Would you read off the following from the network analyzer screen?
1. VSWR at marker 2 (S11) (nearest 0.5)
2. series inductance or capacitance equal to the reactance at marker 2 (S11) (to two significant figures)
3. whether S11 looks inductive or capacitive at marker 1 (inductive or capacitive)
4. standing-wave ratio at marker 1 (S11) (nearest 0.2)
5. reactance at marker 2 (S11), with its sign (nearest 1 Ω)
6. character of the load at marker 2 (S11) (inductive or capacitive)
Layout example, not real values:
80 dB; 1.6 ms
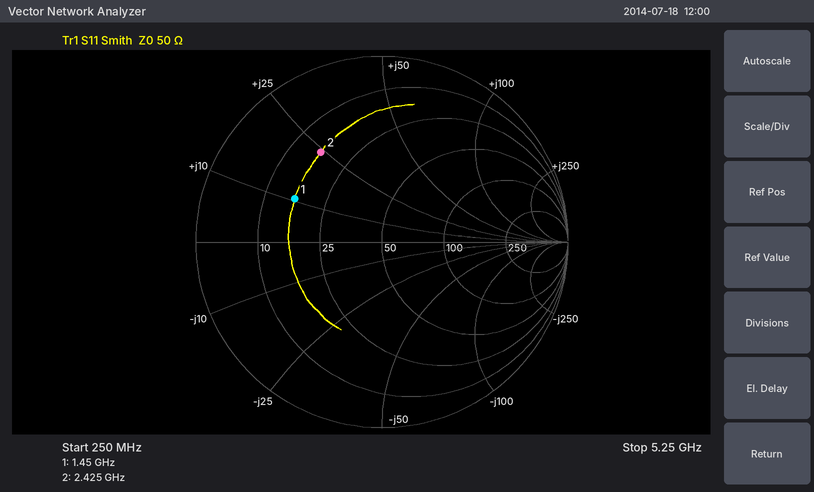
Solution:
4.0; 1.6 nH; inductive; 3.2; +24 Ω; inductive
